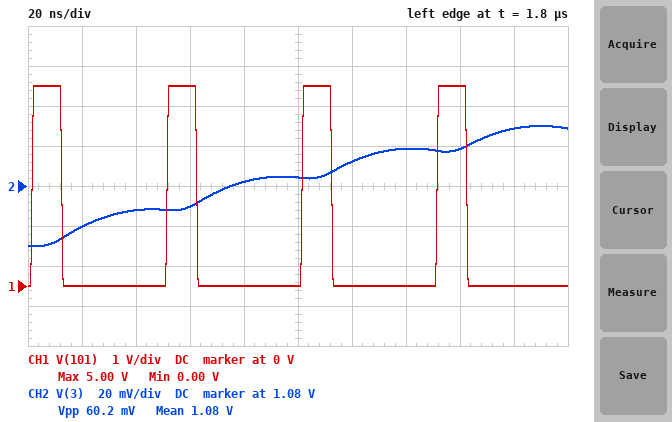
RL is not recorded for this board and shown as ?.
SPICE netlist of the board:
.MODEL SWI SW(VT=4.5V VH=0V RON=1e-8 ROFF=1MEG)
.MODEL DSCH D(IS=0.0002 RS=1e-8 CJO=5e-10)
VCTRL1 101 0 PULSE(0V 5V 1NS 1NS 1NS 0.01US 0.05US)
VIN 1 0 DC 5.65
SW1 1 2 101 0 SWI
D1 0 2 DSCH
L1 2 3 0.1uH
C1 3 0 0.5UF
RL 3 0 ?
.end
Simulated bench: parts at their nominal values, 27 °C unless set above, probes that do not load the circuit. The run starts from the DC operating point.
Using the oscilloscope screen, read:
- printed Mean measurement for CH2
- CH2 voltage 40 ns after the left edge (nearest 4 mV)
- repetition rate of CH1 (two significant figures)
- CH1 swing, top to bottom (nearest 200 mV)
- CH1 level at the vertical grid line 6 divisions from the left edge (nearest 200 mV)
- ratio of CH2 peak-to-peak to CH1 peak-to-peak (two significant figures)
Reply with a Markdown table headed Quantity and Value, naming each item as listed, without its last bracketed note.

| Quantity | Value |
|---|---|
| printed Mean measurement for CH2 | 1.08 V |
| CH2 voltage 40 ns after the left edge | 1.068 V |
| repetition rate of CH1 | 20 MHz |
| CH1 swing, top to bottom | 5.0 V |
| CH1 level at the vertical grid line 6 divisions from the left edge | 0 V |
| ratio of CH2 peak-to-peak to CH1 peak-to-peak | 0.012 |
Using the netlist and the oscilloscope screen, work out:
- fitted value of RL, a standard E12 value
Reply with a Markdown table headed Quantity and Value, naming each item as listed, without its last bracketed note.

| Quantity | Value |
|---|---|
| fitted value of RL, a standard E12 value | 1.5 Ω |
